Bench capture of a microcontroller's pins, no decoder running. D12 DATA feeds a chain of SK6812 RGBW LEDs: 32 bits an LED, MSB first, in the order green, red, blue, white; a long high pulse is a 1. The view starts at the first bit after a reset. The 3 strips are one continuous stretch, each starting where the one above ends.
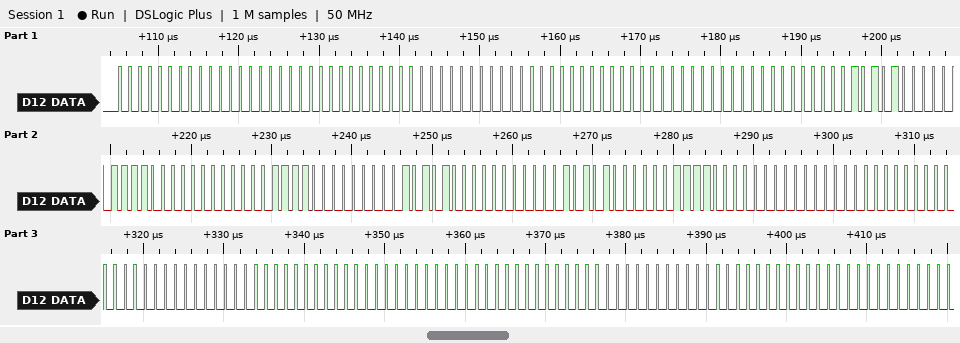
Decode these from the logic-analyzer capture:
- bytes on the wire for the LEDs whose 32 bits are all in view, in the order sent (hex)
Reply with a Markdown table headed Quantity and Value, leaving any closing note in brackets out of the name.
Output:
| Quantity | Value |
|---|---|
| bytes on the wire for the LEDs whose 32 bits are all in view, in the order sent | 00 00 00 00 00 00 00 00 00 54 0F 00 0F 00 54 00 54 0F 00 00 00 00 00 00 00 00 00 00 |
